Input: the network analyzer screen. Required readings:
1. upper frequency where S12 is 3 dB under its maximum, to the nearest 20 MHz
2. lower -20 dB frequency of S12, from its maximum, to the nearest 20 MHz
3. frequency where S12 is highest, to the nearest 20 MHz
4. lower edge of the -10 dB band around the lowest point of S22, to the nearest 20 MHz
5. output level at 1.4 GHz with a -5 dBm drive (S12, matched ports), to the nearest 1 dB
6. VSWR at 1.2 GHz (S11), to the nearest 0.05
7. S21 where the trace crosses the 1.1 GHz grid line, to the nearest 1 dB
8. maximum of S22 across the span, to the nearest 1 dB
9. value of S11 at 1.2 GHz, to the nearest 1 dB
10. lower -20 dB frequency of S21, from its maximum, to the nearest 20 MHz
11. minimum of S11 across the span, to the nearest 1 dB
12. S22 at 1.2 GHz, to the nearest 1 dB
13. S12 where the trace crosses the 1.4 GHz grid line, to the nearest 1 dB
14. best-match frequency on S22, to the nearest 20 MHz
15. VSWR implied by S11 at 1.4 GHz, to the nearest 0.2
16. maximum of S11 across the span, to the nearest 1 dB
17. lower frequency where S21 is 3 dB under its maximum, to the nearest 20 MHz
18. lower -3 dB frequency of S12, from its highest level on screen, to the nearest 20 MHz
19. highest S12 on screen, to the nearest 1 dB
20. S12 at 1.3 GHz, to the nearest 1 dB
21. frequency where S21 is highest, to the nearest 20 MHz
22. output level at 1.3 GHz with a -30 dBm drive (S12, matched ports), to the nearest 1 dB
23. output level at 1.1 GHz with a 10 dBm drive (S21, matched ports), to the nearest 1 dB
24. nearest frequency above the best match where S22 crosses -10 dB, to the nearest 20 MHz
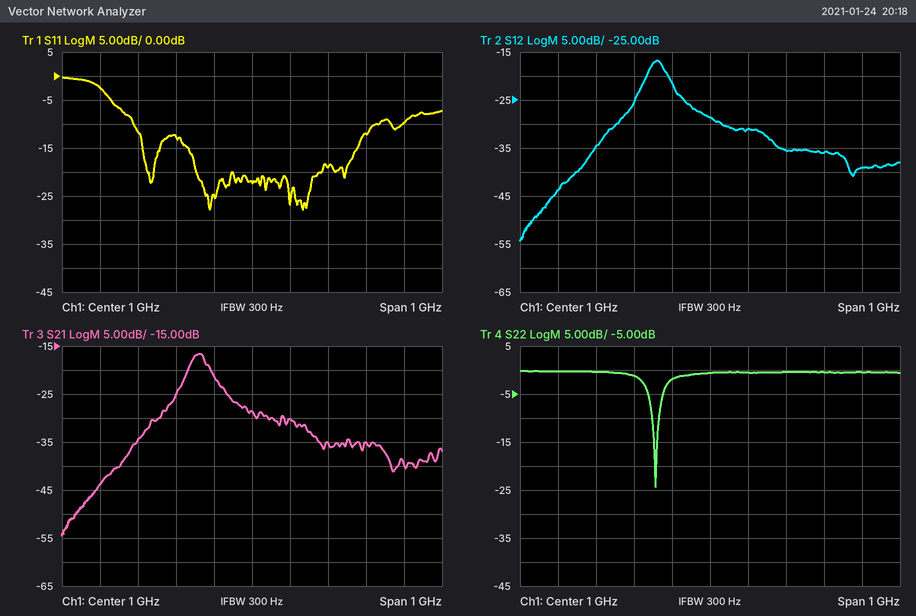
880 MHz
680 MHz
860 MHz
840 MHz
-44 dBm
1.25
-30 dB
0 dB
-19 dB
680 MHz
-28 dB
0 dB
-39 dB
860 MHz
2.0
0 dB
840 MHz
840 MHz
-17 dB
-36 dB
860 MHz
-66 dBm
-20 dBm
860 MHz
